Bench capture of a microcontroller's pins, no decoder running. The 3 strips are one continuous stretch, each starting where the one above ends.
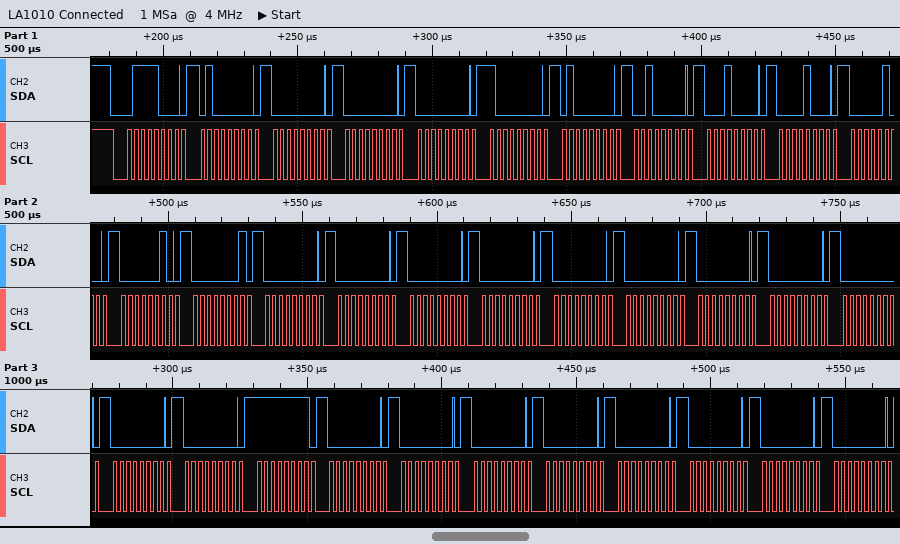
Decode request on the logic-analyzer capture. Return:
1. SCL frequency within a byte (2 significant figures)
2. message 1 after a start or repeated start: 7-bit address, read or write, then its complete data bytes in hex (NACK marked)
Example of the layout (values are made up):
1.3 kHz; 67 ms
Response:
400 kHz; 0x3C write: 40 00 00 00 80 40 20 10 08 04 02 01 00 00 00 00 00 00 00 00 00 00 00 FF 00 00 00 00 00 00 00 00
